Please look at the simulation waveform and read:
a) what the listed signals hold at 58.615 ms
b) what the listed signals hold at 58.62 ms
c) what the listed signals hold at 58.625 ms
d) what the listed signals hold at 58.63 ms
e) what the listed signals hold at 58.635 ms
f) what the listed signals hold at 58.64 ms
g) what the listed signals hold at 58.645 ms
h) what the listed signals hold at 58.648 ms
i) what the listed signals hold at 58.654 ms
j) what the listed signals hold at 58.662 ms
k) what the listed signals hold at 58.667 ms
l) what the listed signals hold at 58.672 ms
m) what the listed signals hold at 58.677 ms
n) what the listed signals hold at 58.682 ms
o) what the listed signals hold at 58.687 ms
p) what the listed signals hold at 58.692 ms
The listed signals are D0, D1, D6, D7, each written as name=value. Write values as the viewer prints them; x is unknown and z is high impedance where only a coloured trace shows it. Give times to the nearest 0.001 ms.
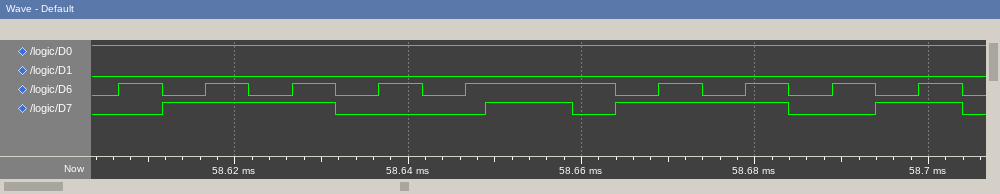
D0=1, D1=0, D6=0, D7=1
D0=1, D1=0, D6=1, D7=1
D0=1, D1=0, D6=0, D7=1
D0=1, D1=0, D6=1, D7=1
D0=1, D1=0, D6=0, D7=0
D0=1, D1=0, D6=1, D7=0
D0=1, D1=0, D6=0, D7=0
D0=1, D1=0, D6=1, D7=0
D0=1, D1=0, D6=1, D7=1
D0=1, D1=0, D6=1, D7=0
D0=1, D1=0, D6=0, D7=1
D0=1, D1=0, D6=1, D7=1
D0=1, D1=0, D6=0, D7=1
D0=1, D1=0, D6=1, D7=1
D0=1, D1=0, D6=0, D7=0
D0=1, D1=0, D6=1, D7=0
